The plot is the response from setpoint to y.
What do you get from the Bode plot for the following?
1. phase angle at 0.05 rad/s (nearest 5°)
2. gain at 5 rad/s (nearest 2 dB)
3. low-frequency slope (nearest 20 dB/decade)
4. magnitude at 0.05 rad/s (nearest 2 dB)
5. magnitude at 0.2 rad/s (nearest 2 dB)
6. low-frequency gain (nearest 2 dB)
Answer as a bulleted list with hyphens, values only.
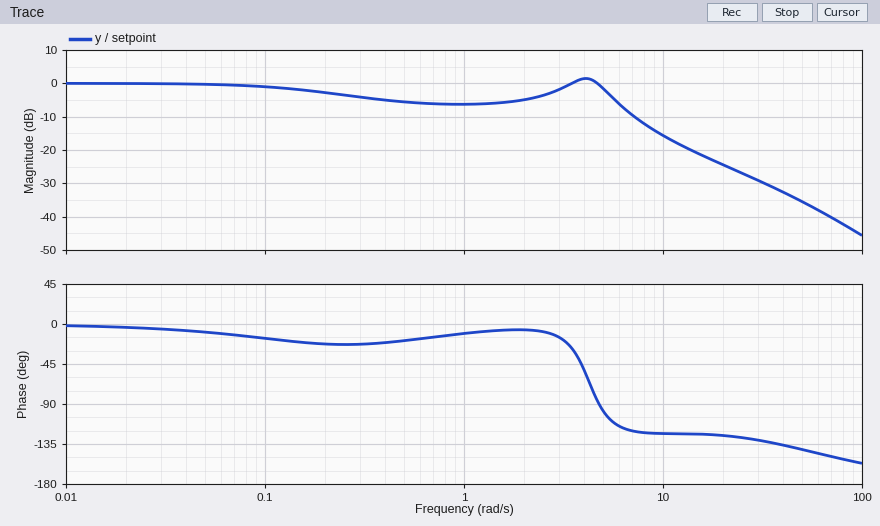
- -10°
- -2 dB
- 0 dB/decade
- 0 dB
- -2 dB
- 0 dB
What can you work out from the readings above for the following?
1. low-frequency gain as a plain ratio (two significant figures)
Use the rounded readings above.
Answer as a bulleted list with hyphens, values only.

- 1.0
